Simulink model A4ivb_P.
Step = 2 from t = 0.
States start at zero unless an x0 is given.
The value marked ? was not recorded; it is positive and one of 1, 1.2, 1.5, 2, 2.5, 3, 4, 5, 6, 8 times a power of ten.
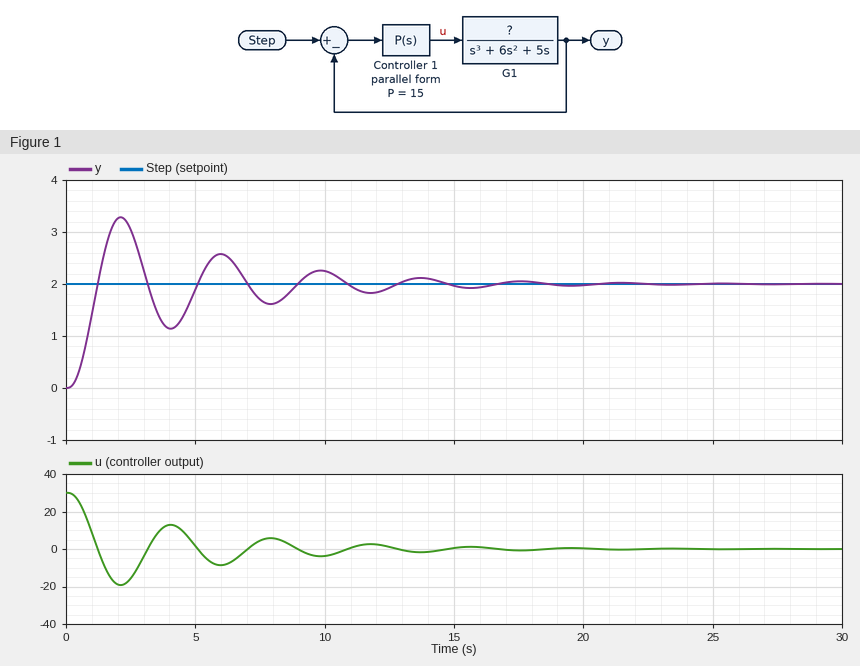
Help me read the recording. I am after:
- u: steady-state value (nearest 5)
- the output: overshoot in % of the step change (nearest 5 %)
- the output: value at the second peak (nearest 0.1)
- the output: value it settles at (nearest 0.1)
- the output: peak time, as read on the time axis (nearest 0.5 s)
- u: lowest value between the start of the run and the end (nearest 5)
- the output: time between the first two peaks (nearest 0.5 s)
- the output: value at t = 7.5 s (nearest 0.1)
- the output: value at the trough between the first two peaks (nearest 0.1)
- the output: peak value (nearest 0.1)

0
65 %
2.6
2.0
2.0 s
-20
4.0 s
1.7
1.1
3.3
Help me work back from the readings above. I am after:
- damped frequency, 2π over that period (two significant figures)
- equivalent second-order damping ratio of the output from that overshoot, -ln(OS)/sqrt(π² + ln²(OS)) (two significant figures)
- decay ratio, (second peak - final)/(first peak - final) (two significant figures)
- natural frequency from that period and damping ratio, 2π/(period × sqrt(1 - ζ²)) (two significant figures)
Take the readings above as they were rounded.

1.6 rad/s
0.14
0.46
1.6 rad/s
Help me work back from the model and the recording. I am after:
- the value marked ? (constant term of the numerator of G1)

1
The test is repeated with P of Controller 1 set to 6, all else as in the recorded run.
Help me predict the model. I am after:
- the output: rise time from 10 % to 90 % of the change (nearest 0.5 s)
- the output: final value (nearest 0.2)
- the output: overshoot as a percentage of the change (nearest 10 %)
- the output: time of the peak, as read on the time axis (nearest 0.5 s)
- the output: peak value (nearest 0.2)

1.5 s
2.0
30 %
3.5 s
2.6
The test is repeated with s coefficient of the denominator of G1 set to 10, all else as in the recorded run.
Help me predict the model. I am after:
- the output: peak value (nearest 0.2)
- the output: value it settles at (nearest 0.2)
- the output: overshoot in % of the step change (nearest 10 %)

2.4
2.0
20 %
